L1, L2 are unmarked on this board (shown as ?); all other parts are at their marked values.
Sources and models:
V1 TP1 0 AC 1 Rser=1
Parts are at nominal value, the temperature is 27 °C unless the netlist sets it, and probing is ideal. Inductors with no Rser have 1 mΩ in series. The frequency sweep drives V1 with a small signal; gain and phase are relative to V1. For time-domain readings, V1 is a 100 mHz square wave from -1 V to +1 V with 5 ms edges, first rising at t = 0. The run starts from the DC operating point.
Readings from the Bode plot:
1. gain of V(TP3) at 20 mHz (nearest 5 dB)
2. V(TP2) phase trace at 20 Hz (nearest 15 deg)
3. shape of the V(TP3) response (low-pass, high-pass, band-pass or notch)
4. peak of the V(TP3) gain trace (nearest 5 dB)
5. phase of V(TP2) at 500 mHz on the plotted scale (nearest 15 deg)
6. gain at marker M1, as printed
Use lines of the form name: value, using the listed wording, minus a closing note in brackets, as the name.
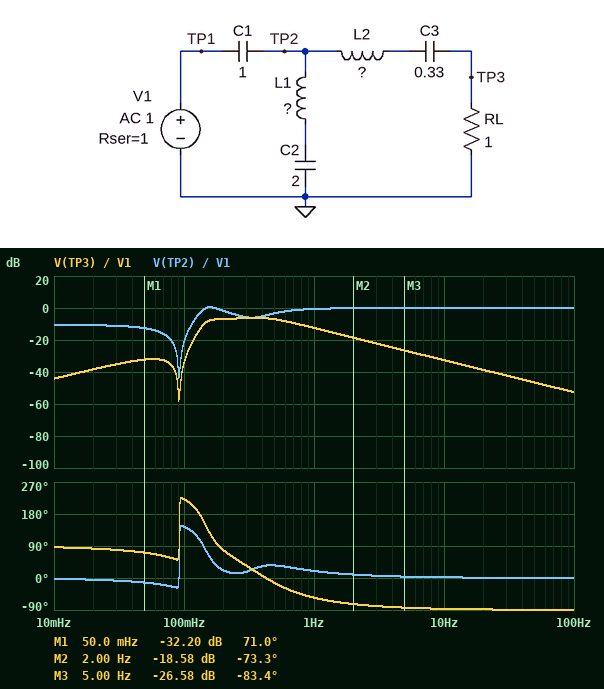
gain of V(TP3) at 20 mHz: -40 dB
V(TP2) phase trace at 20 Hz: 0 deg
shape of the V(TP3) response: band-pass
peak of the V(TP3) gain trace: -5 dB
phase of V(TP2) at 500 mHz on the plotted scale: 30 deg
gain at marker M1, as printed: -32.20 dB
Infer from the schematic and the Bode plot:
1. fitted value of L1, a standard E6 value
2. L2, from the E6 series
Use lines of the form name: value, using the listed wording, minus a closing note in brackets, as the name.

fitted value of L1, a standard E6 value: 1.5 H
L2, from the E6 series: 680 mH
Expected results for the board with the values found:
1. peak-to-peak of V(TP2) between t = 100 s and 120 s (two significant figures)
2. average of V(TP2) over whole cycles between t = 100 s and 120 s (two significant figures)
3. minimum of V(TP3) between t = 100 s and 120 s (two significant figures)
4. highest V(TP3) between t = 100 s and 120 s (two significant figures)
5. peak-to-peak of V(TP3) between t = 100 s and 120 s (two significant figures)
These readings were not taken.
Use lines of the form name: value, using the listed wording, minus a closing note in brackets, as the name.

peak-to-peak of V(TP2) between t = 100 s and 120 s: 3.1 V
average of V(TP2) over whole cycles between t = 100 s and 120 s: 300 mV
minimum of V(TP3) between t = 100 s and 120 s: -400 mV
highest V(TP3) between t = 100 s and 120 s: 400 mV
peak-to-peak of V(TP3) between t = 100 s and 120 s: 800 mV
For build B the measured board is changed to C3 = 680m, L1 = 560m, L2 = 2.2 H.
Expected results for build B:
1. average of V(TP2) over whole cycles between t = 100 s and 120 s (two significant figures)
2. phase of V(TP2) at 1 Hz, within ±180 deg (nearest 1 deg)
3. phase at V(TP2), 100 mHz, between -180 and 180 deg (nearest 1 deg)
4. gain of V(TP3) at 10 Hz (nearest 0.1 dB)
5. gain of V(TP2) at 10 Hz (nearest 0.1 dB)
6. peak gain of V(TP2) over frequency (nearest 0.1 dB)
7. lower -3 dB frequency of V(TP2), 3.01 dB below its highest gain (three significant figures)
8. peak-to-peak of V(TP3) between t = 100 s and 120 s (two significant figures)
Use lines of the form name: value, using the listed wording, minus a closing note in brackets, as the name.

average of V(TP2) over whole cycles between t = 100 s and 120 s: 270 mV
phase of V(TP2) at 1 Hz, within ±180 deg: 21 deg
phase at V(TP2), 100 mHz, between -180 and 180 deg: -18 deg
gain of V(TP3) at 10 Hz: -42.8 dB
gain of V(TP2) at 10 Hz: 0 dB
peak gain of V(TP2) over frequency: 0 dB
lower -3 dB frequency of V(TP2), 3.01 dB below its highest gain: 332 mHz
peak-to-peak of V(TP3) between t = 100 s and 120 s: 470 mV
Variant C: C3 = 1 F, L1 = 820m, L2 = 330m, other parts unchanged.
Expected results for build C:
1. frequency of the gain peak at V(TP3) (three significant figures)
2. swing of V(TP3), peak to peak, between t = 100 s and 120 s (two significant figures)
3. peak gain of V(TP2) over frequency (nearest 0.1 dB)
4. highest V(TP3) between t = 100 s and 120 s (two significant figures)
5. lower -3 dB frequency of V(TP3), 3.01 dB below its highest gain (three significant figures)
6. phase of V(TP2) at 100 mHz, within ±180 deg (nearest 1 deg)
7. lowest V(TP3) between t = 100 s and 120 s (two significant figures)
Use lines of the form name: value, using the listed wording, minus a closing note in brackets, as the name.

frequency of the gain peak at V(TP3): 309 mHz
swing of V(TP3), peak to peak, between t = 100 s and 120 s: 1.1 V
peak gain of V(TP2) over frequency: 0 dB
highest V(TP3) between t = 100 s and 120 s: 550 mV
lower -3 dB frequency of V(TP3), 3.01 dB below its highest gain: 174 mHz
phase of V(TP2) at 100 mHz, within ±180 deg: -24 deg
lowest V(TP3) between t = 100 s and 120 s: -550 mV
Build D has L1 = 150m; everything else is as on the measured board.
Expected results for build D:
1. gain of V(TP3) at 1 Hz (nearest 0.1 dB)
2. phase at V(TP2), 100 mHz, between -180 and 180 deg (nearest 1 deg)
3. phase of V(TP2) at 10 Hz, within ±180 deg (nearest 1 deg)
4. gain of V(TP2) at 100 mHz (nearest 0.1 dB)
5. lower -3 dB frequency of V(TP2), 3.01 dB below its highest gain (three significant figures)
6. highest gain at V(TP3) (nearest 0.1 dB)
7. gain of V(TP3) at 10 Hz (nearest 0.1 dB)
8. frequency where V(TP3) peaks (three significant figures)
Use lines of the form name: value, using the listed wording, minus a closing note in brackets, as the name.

gain of V(TP3) at 1 Hz: -16.2 dB
phase at V(TP2), 100 mHz, between -180 and 180 deg: -23 deg
phase of V(TP2) at 10 Hz, within ±180 deg: 7 deg
gain of V(TP2) at 100 mHz: -12.0 dB
lower -3 dB frequency of V(TP2), 3.01 dB below its highest gain: 1.26 Hz
highest gain at V(TP3): -15.2 dB
gain of V(TP3) at 10 Hz: -32.7 dB
frequency where V(TP3) peaks: 600 mHz
